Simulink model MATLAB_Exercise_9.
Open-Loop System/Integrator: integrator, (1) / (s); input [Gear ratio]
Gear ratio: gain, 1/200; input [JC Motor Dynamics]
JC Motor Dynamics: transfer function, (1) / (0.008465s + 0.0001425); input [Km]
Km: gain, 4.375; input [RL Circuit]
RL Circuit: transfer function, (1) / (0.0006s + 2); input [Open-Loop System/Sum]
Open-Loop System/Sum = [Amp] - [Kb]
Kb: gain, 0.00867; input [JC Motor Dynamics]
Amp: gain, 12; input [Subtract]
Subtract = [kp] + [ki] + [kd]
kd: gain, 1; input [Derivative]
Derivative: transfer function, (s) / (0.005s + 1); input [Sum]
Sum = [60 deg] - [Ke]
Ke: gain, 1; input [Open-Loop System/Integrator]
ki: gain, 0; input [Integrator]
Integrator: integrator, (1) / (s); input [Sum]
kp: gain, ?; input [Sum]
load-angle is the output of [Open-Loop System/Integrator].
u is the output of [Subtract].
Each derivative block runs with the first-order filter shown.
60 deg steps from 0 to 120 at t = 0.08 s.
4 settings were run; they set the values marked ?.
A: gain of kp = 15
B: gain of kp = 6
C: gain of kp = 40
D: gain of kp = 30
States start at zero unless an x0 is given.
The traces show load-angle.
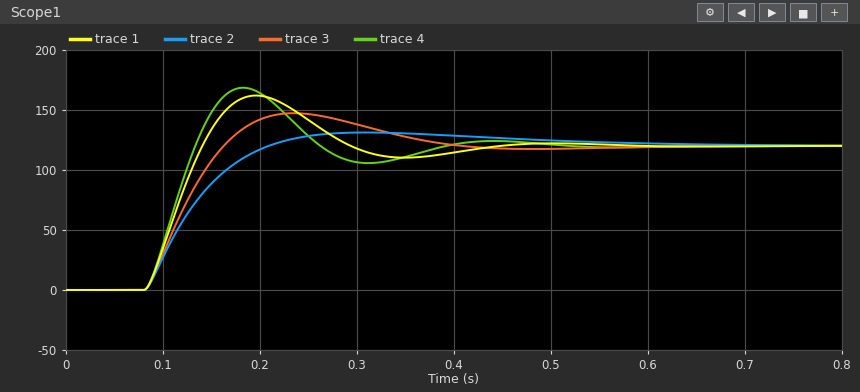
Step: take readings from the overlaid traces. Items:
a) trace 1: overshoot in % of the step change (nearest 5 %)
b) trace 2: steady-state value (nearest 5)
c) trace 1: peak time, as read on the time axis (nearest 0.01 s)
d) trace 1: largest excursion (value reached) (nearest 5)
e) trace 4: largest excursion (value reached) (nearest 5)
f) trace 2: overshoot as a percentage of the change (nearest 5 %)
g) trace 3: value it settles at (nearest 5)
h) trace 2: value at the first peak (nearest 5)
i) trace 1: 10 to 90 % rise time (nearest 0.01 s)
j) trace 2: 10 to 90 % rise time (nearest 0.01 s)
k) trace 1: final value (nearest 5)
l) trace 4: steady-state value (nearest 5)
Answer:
35 %
120
0.20 s
160
170
10 %
120
130
0.04 s
0.09 s
120
120
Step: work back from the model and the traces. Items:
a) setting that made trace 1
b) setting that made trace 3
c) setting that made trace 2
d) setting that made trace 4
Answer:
D
A
B
C
